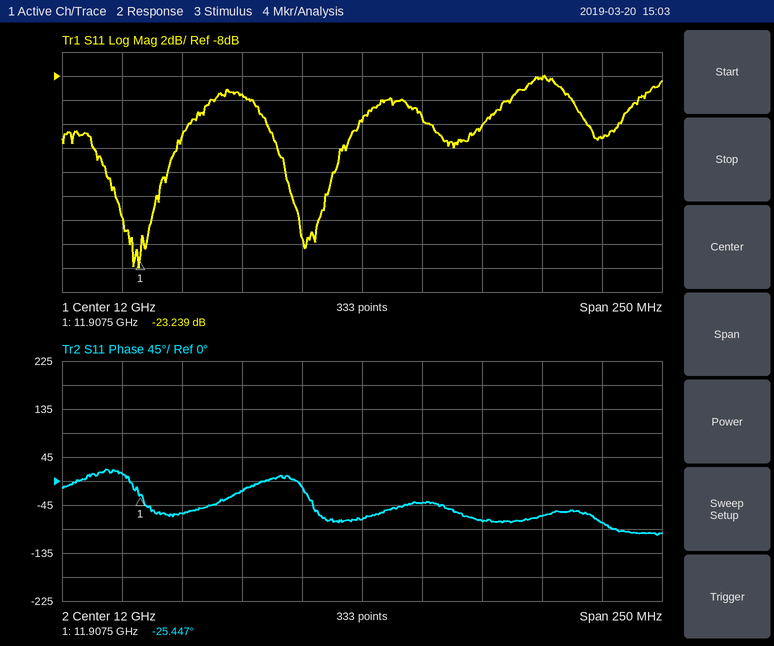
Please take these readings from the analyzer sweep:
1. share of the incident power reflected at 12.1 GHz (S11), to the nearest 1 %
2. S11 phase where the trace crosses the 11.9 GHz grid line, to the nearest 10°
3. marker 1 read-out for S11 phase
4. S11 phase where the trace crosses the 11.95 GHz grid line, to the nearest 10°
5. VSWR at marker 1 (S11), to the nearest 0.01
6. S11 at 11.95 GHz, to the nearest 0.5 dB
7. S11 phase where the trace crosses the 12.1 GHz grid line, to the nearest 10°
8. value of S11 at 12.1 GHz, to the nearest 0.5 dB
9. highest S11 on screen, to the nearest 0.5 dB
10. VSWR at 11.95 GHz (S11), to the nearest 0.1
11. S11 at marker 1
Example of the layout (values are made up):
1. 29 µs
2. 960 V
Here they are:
1. 5 %
2. 10°
3. -25.447°
4. -20°
5. 1.15
6. -9.5 dB
7. -80°
8. -13.0 dB
9. -8.0 dB
10. 2.0
11. -23.239 dB
